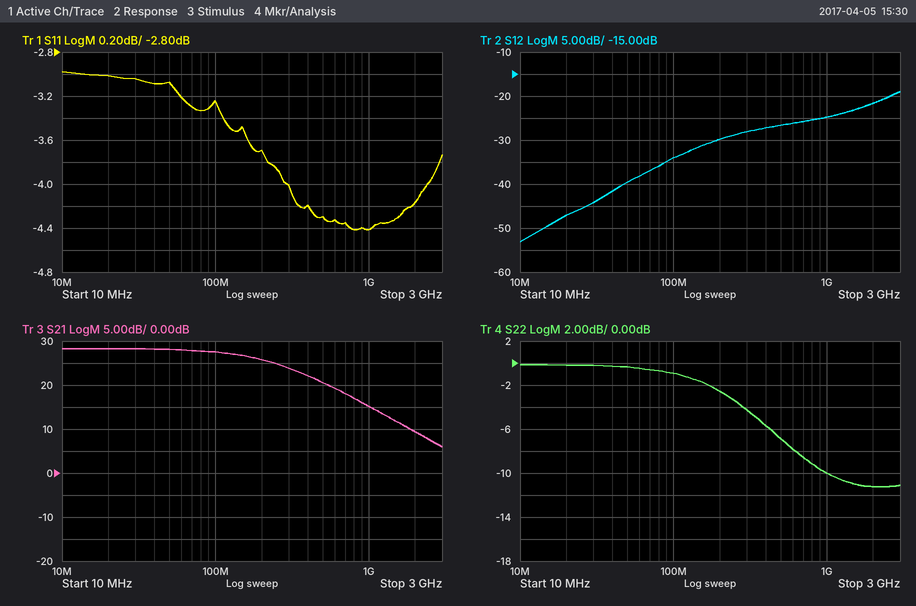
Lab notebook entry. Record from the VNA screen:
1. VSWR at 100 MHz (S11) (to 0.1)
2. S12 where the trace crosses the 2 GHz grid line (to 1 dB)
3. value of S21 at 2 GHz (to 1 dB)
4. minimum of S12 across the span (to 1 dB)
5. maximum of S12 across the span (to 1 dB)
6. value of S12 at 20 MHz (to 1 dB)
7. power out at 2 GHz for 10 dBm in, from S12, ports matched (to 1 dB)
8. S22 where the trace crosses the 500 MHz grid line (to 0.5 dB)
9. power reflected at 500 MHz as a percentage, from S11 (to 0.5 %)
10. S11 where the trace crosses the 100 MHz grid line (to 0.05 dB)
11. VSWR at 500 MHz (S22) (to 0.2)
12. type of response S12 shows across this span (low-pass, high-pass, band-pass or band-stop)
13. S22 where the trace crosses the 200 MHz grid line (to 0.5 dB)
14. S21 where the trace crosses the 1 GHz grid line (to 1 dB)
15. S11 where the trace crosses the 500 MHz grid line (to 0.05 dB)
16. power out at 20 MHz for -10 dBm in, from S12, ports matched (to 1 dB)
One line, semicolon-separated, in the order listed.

5.4; -22 dB; 9 dB; -53 dB; -19 dB; -47 dB; -12 dBm; -7.0 dB; 37.0 %; -3.25 dB; 2.6; high-pass; -2.5 dB; 15 dB; -4.30 dB; -57 dBm
